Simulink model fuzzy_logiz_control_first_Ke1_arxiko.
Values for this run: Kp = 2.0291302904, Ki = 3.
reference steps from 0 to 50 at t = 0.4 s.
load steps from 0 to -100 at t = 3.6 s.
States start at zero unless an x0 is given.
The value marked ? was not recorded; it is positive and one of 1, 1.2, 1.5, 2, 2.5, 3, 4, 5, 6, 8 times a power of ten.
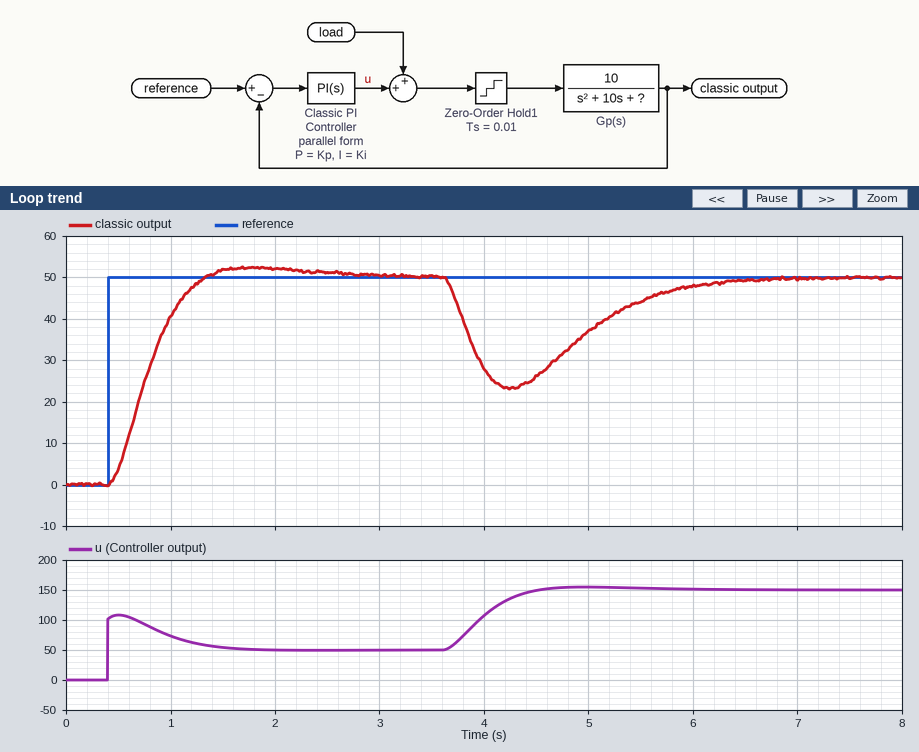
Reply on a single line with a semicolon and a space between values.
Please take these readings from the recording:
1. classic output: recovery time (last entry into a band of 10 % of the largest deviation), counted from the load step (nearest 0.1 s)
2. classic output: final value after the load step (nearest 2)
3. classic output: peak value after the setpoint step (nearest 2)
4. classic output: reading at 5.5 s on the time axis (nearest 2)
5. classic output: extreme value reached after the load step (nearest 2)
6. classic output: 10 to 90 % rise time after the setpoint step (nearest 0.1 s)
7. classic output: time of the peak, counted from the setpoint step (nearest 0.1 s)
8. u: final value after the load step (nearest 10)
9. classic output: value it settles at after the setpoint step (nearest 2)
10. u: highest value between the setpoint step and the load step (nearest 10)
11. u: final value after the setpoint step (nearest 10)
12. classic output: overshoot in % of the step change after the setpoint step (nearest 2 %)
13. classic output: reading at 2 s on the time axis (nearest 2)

2.3 s; 50; 52; 44; 24; 0.6 s; 1.4 s; 150; 50; 110; 50; 4 %; 52
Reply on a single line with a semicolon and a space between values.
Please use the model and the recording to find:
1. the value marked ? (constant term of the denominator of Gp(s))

10
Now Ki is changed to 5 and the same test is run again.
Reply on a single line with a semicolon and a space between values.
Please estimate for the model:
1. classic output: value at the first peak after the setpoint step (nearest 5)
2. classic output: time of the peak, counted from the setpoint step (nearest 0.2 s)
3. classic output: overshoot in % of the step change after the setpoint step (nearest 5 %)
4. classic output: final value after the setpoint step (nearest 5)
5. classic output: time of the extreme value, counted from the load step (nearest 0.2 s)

60; 1.0 s; 20 %; 50; 0.6 s
